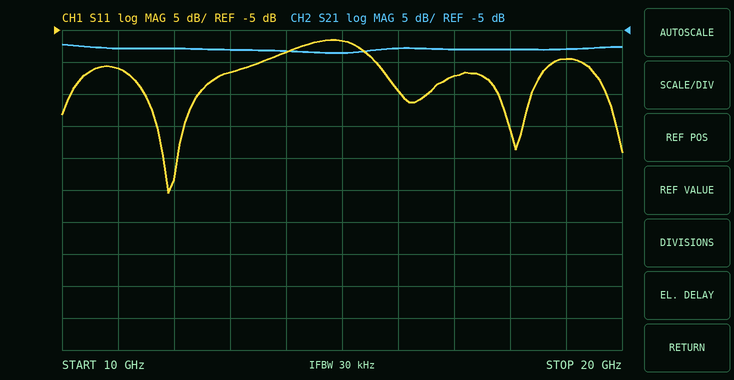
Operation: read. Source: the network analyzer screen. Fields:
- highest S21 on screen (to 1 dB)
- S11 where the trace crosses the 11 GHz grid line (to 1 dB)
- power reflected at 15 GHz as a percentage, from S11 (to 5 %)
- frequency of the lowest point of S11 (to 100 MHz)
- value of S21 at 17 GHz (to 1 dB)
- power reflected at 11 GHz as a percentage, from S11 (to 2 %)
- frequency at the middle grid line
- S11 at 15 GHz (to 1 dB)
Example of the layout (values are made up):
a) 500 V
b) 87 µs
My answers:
a) -7 dB
b) -11 dB
c) 20 %
d) 11.9 GHz
e) -8 dB
f) 8 %
g) 15 GHz
h) -7 dB
